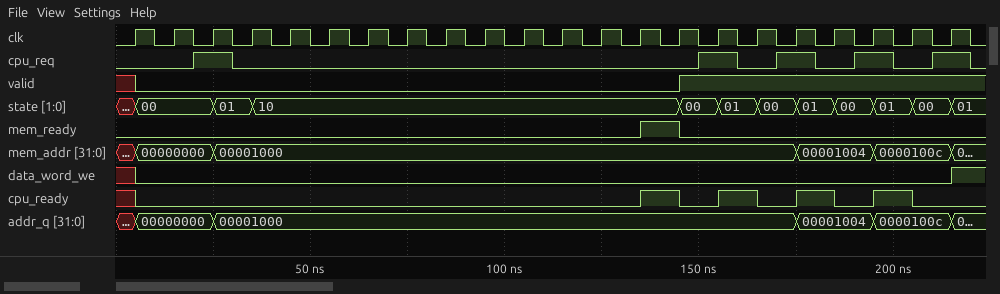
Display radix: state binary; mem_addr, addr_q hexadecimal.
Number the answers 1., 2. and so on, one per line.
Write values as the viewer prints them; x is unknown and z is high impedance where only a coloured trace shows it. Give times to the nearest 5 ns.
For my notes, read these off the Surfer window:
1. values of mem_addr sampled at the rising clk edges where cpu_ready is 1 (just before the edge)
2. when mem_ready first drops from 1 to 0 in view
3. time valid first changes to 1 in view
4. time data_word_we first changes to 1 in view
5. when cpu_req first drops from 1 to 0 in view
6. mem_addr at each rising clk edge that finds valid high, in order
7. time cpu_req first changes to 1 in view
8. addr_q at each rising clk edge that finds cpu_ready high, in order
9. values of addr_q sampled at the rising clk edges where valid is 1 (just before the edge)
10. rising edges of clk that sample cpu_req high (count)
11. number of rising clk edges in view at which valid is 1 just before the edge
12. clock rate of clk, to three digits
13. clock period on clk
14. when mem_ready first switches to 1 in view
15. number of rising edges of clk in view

1. 00001000, 00001000, 00001004, 0000100c
2. 145 ns
3. 145 ns
4. 215 ns
5. 30 ns
6. 00001000, 00001000, 00001000, 00001004, 00001004, 0000100c, 0000100c
7. 20 ns
8. 00001000, 00001000, 00001004, 0000100c
9. 00001000, 00001000, 00001000, 00001004, 00001004, 0000100c, 0000100c
10. 5
11. 7
12. 100 MHz
13. 10 ns
14. 135 ns
15. 22
